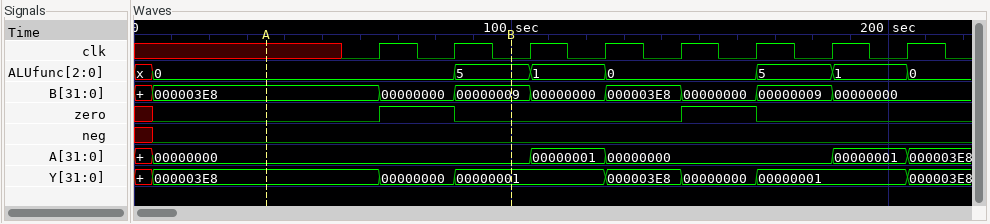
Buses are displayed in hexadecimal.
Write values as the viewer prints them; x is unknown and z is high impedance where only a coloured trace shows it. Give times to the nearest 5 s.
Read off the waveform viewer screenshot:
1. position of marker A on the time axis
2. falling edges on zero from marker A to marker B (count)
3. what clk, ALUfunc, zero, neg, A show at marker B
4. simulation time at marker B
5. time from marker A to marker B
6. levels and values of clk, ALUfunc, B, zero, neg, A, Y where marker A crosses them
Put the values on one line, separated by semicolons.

35 s; 1; clk=0, ALUfunc=5, zero=0, neg=0, A=00000000; 100 s; 65 s; clk=x, ALUfunc=0, B=000003E8, zero=0, neg=0, A=00000000, Y=000003E8
